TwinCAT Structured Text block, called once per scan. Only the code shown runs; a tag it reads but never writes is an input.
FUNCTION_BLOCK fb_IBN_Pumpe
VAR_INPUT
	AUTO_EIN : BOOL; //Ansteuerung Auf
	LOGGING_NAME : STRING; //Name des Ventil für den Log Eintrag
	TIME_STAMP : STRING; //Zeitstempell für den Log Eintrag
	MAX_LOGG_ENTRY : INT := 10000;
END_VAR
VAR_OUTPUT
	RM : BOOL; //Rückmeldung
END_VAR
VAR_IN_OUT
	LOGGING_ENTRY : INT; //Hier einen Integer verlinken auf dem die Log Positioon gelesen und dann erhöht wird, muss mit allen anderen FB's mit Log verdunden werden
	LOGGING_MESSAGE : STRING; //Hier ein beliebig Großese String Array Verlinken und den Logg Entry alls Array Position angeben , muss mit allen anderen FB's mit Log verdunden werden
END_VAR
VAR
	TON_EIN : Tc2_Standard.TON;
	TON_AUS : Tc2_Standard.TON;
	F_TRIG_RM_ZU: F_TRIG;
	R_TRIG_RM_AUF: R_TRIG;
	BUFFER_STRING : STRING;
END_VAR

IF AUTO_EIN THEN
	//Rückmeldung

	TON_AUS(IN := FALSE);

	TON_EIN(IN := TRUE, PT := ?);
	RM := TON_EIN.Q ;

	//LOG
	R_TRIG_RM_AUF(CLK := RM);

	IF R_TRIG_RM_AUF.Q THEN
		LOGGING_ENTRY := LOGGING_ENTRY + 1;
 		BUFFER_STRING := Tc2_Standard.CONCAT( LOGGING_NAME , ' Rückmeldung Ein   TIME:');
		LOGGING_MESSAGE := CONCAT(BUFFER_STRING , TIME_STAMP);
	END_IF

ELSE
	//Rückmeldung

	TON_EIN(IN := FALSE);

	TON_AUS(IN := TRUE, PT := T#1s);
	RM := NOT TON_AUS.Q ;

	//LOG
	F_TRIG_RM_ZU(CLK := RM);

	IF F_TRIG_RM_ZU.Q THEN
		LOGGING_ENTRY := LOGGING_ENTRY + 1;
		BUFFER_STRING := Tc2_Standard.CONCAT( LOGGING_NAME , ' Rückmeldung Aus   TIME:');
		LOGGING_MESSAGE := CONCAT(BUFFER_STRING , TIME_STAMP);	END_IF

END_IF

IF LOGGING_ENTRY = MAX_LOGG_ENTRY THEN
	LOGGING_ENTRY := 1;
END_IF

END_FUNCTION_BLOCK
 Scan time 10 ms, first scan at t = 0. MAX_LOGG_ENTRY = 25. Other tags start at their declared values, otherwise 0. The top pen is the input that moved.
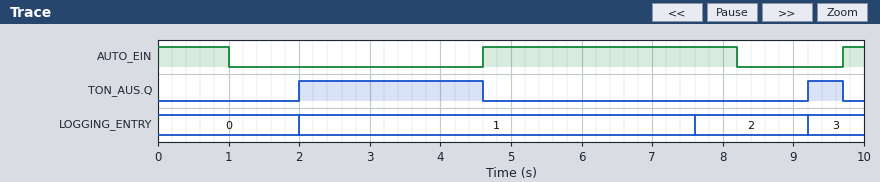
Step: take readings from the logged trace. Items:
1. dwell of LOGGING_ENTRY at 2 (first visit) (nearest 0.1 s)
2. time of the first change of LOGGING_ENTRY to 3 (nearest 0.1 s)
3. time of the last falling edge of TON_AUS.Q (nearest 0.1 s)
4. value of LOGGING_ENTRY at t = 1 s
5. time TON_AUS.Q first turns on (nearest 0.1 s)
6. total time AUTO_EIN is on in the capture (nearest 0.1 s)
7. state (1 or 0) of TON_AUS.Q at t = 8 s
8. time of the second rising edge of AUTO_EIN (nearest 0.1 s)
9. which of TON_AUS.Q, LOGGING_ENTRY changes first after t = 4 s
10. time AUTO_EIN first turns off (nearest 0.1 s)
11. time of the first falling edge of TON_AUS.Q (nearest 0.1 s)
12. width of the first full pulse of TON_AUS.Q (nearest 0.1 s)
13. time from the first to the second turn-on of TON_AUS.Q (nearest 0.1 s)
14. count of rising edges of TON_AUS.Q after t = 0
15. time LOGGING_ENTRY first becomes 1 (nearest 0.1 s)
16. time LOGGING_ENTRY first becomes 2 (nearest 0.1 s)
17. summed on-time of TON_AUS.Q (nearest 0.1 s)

1.6 s
9.2 s
9.7 s
0
2.0 s
4.9 s
0
9.7 s
TON_AUS.Q
1.0 s
4.6 s
2.6 s
7.2 s
2
2.0 s
7.6 s
3.1 s
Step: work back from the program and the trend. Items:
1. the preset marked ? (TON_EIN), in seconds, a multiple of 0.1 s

3.0 s
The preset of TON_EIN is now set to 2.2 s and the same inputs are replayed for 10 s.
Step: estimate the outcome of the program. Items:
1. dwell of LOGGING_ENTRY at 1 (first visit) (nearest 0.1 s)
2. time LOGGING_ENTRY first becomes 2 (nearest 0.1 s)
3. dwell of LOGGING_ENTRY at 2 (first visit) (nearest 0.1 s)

4.8 s
6.8 s
2.4 s
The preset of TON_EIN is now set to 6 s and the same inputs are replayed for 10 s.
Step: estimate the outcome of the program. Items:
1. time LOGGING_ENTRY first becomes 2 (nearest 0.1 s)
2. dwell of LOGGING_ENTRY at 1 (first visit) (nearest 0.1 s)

9.2 s
7.2 s
